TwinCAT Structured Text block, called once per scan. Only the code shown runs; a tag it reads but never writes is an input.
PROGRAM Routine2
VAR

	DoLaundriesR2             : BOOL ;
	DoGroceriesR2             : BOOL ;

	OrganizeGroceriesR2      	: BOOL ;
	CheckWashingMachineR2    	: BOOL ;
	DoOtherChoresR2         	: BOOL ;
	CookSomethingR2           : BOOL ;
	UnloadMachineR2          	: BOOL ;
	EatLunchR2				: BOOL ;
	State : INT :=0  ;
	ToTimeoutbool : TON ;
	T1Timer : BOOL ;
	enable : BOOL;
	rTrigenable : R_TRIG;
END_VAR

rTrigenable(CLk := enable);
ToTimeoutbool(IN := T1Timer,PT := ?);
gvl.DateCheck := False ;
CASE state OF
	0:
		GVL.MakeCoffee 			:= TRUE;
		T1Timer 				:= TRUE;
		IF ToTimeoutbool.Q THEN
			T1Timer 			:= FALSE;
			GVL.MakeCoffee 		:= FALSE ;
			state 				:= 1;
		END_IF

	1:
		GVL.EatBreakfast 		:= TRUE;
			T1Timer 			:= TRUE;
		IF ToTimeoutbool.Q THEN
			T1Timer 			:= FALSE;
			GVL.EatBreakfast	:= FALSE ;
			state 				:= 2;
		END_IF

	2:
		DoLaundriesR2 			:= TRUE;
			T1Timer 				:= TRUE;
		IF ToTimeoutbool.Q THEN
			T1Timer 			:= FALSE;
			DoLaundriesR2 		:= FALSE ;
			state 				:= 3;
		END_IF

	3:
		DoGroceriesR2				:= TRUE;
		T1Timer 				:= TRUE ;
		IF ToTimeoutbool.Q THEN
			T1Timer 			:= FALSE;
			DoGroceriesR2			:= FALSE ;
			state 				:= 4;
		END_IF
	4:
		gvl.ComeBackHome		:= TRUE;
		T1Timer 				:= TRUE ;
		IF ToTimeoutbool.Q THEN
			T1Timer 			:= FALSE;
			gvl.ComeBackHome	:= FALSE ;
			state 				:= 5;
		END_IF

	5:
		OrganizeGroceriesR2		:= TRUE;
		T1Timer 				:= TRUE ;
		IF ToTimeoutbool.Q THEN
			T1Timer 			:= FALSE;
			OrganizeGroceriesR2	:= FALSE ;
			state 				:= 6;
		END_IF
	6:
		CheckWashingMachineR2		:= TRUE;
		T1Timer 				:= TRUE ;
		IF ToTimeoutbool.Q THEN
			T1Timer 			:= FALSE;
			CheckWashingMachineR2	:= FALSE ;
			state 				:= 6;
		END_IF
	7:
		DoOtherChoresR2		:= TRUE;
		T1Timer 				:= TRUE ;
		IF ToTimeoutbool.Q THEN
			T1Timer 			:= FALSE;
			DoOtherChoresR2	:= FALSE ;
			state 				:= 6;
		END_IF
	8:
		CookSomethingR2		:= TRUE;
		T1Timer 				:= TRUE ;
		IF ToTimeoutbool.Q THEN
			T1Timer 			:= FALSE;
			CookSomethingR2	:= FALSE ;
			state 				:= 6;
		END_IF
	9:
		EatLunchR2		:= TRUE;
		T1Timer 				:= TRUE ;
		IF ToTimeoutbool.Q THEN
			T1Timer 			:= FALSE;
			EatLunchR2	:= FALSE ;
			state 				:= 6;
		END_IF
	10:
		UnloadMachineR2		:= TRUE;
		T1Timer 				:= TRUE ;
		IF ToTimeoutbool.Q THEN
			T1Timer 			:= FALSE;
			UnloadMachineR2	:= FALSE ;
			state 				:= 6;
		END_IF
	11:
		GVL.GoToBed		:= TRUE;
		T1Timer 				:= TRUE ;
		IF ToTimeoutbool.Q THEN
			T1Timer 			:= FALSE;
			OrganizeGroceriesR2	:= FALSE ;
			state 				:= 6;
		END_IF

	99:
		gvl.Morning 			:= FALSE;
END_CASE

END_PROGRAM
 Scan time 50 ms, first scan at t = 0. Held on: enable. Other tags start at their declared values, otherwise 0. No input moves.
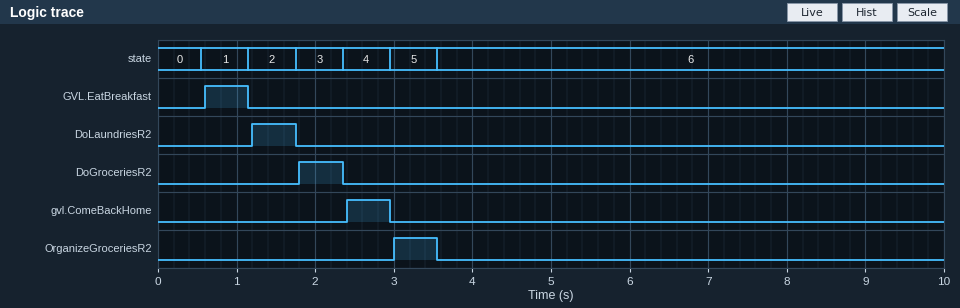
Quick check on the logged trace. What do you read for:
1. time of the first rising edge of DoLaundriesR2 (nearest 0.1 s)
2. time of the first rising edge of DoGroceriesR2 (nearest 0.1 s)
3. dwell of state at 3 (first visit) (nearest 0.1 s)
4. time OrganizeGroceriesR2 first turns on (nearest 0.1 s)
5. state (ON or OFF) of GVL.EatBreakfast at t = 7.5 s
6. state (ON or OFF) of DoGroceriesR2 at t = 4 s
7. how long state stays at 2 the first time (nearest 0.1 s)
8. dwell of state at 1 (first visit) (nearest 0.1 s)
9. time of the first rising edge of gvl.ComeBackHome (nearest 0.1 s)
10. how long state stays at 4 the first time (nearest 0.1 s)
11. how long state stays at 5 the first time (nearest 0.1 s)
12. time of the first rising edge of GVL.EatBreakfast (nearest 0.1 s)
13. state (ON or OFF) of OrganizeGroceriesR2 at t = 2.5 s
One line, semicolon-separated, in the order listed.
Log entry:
1.2 s; 1.8 s; 0.6 s; 3.0 s; OFF; OFF; 0.6 s; 0.6 s; 2.4 s; 0.6 s; 0.6 s; 0.6 s; OFF
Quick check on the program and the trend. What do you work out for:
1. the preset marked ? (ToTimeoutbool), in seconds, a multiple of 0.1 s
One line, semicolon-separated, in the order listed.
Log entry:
0.5 s
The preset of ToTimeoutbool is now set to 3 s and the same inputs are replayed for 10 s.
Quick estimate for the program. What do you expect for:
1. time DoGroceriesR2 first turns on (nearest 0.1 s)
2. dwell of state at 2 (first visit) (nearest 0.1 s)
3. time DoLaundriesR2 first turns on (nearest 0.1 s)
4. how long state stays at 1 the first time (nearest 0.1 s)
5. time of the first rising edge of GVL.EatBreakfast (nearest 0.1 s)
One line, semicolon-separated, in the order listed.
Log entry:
9.3 s; 3.1 s; 6.2 s; 3.1 s; 3.1 s
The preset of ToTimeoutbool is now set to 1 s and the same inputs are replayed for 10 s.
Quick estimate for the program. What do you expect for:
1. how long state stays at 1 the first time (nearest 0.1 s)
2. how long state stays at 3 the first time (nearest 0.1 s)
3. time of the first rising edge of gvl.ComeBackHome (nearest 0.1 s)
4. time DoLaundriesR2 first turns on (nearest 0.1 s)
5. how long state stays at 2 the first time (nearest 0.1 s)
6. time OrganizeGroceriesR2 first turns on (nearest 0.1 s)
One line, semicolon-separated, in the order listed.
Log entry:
1.1 s; 1.1 s; 4.4 s; 2.2 s; 1.1 s; 5.5 s
